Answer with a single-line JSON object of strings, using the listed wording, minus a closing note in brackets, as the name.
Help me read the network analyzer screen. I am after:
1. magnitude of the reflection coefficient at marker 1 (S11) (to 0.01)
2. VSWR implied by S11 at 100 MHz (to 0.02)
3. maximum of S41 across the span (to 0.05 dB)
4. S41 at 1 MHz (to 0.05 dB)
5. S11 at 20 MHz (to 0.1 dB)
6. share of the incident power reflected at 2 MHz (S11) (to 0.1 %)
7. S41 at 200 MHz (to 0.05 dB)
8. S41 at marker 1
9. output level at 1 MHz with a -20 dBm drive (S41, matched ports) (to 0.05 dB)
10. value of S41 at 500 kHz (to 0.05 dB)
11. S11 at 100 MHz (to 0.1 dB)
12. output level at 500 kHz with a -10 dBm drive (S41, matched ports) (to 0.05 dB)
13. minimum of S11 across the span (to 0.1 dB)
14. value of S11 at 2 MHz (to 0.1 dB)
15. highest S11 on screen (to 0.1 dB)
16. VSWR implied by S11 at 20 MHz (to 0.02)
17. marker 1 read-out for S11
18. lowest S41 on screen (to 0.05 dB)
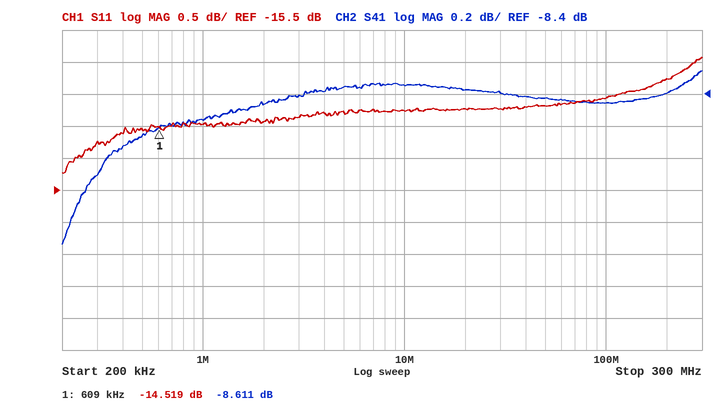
{"magnitude of the reflection coefficient at marker 1 (S11)": "0.19", "VSWR implied by S11 at 100 MHz": "1.50", "maximum of S41 across the span": "-8.25 dB", "S41 at 1 MHz": "-8.55 dB", "S11 at 20 MHz": "-14.2 dB", "share of the incident power reflected at 2 MHz (S11)": "3.6 %", "S41 at 200 MHz": "-8.40 dB", "S41 at marker 1": "-8.611 dB", "output level at 1 MHz with a -20 dBm drive (S41, matched ports)": "-28.55 dBm", "value of S41 at 500 kHz": "-8.65 dB", "S11 at 100 MHz": "-14.1 dB", "output level at 500 kHz with a -10 dBm drive (S41, matched ports)": "-18.65 dBm", "minimum of S11 across the span": "-15.2 dB", "value of S11 at 2 MHz": "-14.4 dB", "highest S11 on screen": "-13.4 dB", "VSWR implied by S11 at 20 MHz": "1.48", "marker 1 read-out for S11": "-14.519 dB", "lowest S41 on screen": "-9.35 dB"}
